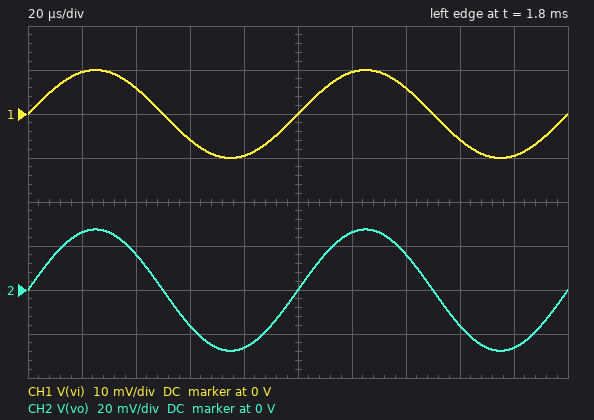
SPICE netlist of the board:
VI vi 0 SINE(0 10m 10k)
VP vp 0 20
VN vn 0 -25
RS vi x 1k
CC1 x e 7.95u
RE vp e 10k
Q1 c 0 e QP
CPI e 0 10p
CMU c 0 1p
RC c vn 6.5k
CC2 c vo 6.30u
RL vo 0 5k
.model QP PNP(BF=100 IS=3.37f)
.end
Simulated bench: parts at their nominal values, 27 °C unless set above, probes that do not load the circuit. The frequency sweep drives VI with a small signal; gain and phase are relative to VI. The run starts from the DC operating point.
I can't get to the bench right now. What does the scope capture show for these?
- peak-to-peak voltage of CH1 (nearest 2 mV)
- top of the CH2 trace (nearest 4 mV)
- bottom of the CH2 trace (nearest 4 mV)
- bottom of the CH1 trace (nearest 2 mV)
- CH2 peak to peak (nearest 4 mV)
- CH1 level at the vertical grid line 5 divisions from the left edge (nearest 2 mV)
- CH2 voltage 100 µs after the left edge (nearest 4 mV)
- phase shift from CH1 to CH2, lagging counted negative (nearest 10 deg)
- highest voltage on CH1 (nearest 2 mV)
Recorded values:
20 mV
28 mV
-28 mV
-10 mV
56 mV
0 V
0 V
0 deg
10 mV
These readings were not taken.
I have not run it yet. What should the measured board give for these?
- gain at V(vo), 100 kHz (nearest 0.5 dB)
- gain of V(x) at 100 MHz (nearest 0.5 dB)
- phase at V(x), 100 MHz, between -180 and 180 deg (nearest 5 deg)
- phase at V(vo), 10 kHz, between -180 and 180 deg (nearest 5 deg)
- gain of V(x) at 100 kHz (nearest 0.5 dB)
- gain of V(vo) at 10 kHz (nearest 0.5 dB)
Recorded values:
9.0 dB
-37.5 dB
-5 deg
0 deg
-37.5 dB
9.0 dB
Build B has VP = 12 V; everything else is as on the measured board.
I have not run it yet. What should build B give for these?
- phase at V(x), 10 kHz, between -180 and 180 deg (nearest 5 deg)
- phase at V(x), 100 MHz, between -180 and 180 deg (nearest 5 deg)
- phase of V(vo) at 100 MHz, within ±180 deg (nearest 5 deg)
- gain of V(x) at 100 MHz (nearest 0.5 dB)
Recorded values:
-5 deg
-10 deg
-70 deg
-33.0 dB
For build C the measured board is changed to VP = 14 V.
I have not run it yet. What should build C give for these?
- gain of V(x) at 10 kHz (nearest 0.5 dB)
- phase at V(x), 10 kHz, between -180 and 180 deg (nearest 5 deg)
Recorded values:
-34.5 dB
-5 deg
